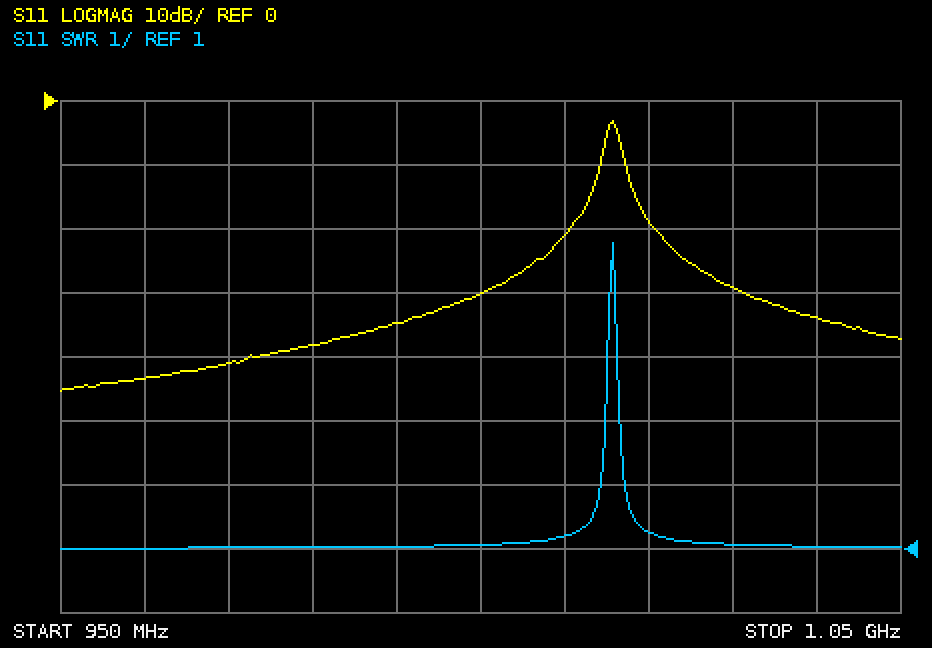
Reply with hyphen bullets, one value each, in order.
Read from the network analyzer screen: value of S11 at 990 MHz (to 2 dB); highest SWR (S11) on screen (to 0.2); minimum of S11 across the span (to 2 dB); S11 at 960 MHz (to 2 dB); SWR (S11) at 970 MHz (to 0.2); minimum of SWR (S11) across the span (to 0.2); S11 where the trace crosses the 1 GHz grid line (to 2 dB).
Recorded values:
- -34 dB
- 5.8
- -46 dB
- -44 dB
- 1.0
- 1.0
- -30 dB
